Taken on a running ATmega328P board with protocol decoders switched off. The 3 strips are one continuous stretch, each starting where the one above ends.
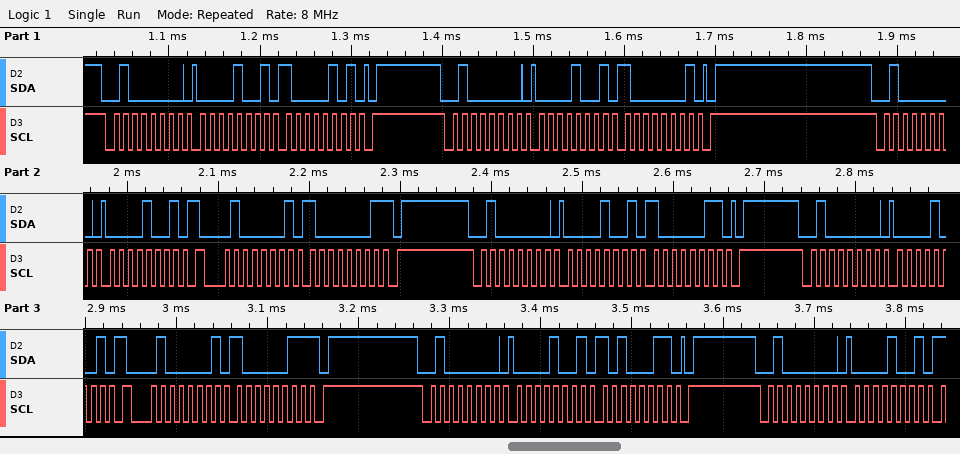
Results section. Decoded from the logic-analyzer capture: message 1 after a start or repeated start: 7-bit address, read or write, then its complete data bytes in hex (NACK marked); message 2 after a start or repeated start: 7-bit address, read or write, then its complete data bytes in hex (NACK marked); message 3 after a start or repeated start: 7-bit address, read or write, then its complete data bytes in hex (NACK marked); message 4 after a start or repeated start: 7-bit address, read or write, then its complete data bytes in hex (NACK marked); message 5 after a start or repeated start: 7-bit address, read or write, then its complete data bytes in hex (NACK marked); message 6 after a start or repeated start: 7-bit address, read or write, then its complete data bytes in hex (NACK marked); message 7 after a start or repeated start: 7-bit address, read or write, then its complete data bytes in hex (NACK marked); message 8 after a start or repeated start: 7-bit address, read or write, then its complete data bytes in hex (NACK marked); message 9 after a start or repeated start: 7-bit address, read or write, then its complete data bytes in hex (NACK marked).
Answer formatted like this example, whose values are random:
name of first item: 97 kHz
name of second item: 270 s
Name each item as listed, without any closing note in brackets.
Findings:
message 1 after a start or repeated start: 7-bit address, read or write, then its complete data bytes in hex: 0x20 write: 09 85
message 2 after a start or repeated start: 7-bit address, read or write, then its complete data bytes in hex: 0x20 write: 09 81
message 3 after a start or repeated start: 7-bit address, read or write, then its complete data bytes in hex: 0x20 write: 09
message 4 after a start or repeated start: 7-bit address, read or write, then its complete data bytes in hex: 0x20 read: 81 NACK
message 5 after a start or repeated start: 7-bit address, read or write, then its complete data bytes in hex: 0x20 write: 09 83
message 6 after a start or repeated start: 7-bit address, read or write, then its complete data bytes in hex: 0x20 write: 09
message 7 after a start or repeated start: 7-bit address, read or write, then its complete data bytes in hex: 0x20 read: 83 NACK
message 8 after a start or repeated start: 7-bit address, read or write, then its complete data bytes in hex: 0x20 write: 09 A3
message 9 after a start or repeated start: 7-bit address, read or write, then its complete data bytes in hex: 0x20 write: 09
